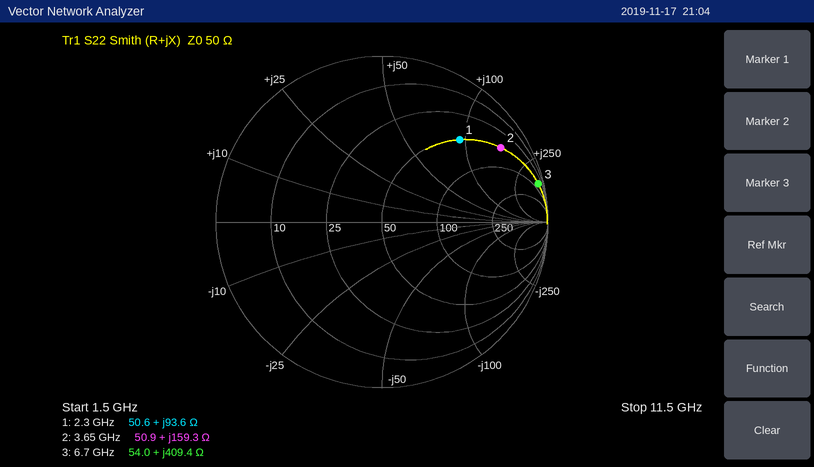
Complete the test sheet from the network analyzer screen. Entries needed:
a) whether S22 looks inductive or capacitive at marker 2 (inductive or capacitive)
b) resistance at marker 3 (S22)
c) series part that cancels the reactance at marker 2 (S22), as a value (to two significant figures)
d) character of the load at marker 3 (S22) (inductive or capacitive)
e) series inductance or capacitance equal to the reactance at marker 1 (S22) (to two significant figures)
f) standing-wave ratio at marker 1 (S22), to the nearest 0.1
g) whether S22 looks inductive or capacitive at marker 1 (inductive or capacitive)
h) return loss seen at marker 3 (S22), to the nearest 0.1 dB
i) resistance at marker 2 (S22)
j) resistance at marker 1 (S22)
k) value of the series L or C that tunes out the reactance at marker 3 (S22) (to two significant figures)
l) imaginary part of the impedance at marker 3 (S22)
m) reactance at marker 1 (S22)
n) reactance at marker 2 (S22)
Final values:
inductive
54.0 Ω
270 fF
inductive
6.5 nH
5.3
inductive
0.3 dB
50.9 Ω
50.6 Ω
58 fF
+409.4 Ω
+93.6 Ω
+159.3 Ω
